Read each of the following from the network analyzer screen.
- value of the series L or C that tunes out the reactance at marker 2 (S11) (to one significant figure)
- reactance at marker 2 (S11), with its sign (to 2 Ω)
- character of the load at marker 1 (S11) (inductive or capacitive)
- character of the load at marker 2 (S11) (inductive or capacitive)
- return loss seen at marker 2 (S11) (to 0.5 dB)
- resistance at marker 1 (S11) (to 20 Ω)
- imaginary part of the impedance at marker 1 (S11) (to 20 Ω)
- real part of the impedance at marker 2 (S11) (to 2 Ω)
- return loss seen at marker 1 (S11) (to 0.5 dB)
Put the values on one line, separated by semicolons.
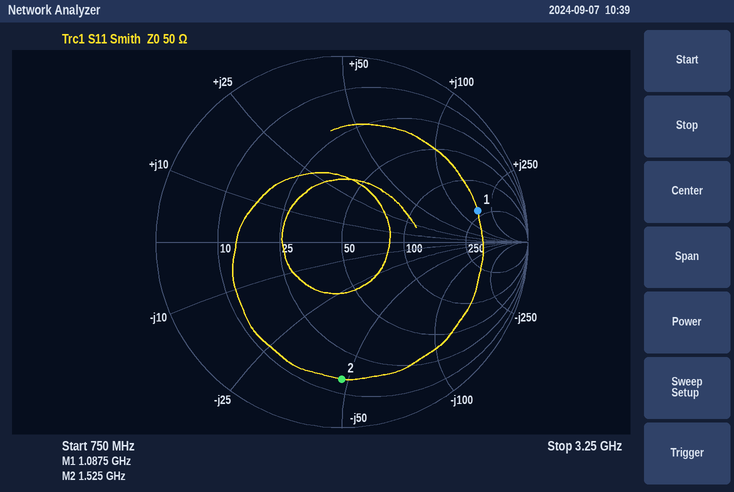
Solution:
5 nH; -48 Ω; inductive; capacitive; 2.5 dB; 220 Ω; +160 Ω; 14 Ω; 2.5 dB
